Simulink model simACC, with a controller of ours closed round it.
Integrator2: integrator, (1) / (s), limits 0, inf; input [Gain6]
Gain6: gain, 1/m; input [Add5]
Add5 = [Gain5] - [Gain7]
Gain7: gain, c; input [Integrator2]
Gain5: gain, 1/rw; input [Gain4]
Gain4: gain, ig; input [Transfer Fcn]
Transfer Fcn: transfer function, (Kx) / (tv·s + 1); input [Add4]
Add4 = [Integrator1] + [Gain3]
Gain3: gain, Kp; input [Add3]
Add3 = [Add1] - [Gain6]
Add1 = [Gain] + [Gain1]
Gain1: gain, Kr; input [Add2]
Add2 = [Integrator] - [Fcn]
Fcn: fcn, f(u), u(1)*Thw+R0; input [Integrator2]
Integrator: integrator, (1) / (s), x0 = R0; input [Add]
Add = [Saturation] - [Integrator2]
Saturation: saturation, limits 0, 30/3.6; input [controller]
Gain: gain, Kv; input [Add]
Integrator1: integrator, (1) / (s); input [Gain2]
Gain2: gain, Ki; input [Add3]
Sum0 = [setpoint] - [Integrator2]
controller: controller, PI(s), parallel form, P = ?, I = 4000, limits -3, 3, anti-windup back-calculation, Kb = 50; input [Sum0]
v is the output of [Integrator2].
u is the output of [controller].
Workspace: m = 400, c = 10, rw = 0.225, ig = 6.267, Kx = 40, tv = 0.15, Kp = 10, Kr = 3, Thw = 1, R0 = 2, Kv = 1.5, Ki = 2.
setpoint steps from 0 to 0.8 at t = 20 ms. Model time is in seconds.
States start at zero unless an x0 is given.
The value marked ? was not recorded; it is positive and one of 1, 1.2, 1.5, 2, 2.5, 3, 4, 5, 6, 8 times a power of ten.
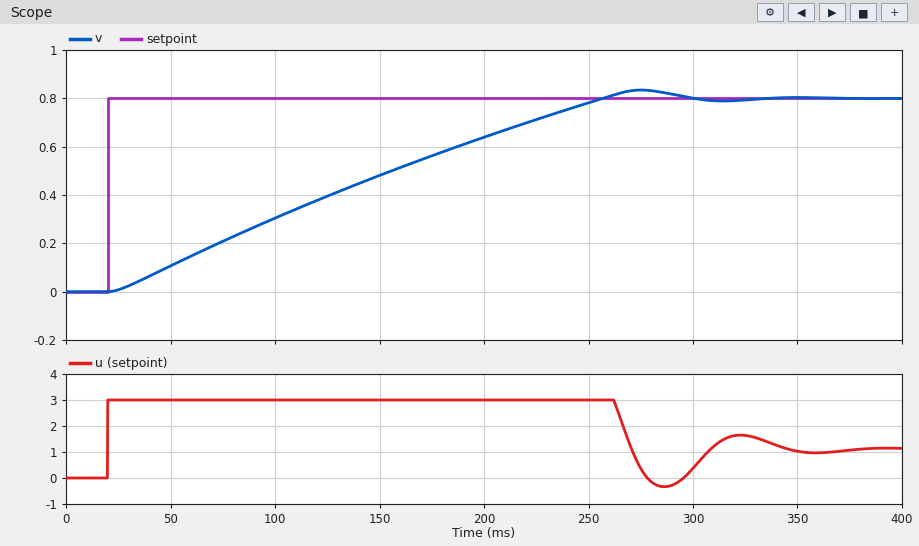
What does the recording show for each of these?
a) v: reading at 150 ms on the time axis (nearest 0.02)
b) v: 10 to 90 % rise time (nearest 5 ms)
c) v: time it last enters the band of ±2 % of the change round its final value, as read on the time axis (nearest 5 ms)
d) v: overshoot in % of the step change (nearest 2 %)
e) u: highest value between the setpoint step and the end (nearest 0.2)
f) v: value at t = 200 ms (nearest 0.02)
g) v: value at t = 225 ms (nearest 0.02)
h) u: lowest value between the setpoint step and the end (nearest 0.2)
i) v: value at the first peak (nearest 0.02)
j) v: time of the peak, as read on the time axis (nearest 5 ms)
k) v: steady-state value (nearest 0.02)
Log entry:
0.48
185 ms
290 ms
4 %
3.0
0.64
0.72
-0.4
0.84
275 ms
0.80
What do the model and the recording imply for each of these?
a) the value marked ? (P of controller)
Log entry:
60
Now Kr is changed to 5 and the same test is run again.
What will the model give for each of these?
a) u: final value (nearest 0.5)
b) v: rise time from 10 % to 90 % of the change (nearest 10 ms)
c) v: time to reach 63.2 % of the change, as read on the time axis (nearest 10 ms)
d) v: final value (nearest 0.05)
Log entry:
1.0
190 ms
160 ms
0.80
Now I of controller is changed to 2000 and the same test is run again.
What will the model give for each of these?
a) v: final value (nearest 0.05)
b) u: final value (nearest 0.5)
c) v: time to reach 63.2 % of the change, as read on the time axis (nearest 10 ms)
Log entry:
0.80
1.0
160 ms
